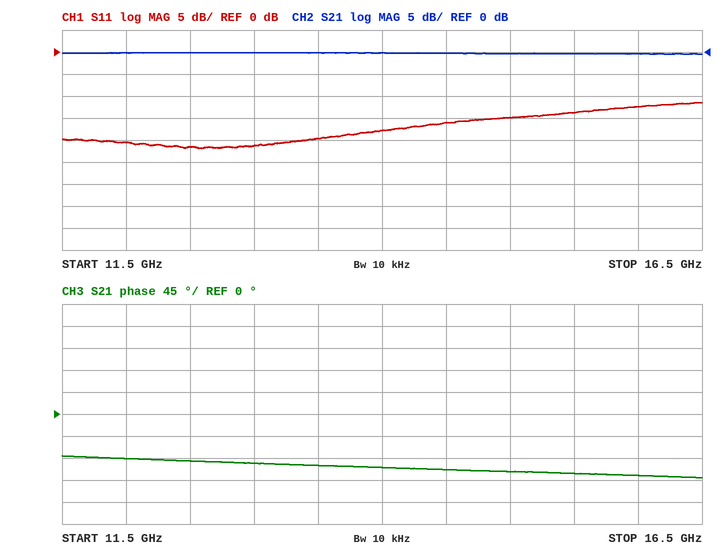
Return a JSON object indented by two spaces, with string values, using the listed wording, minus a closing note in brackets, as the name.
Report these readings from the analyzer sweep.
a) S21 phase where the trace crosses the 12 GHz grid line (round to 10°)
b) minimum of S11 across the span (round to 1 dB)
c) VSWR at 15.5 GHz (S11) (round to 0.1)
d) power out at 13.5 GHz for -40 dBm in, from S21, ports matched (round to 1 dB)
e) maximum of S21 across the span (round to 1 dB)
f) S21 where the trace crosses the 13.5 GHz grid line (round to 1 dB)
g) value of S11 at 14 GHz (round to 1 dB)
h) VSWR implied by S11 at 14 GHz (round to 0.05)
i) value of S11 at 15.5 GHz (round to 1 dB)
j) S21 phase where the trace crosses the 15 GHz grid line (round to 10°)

{
  "S21 phase where the trace crosses the 12 GHz grid line": "-90°",
  "minimum of S11 across the span": "-22 dB",
  "VSWR at 15.5 GHz (S11)": "1.5",
  "power out at 13.5 GHz for -40 dBm in, from S21, ports matched": "-40 dBm",
  "maximum of S21 across the span": "0 dB",
  "S21 where the trace crosses the 13.5 GHz grid line": "0 dB",
  "value of S11 at 14 GHz": "-18 dB",
  "VSWR implied by S11 at 14 GHz": "1.30",
  "value of S11 at 15.5 GHz": "-14 dB",
  "S21 phase where the trace crosses the 15 GHz grid line": "-120°"
}
